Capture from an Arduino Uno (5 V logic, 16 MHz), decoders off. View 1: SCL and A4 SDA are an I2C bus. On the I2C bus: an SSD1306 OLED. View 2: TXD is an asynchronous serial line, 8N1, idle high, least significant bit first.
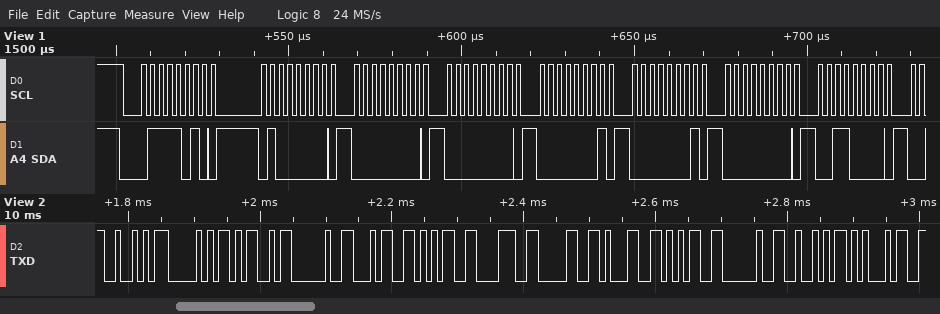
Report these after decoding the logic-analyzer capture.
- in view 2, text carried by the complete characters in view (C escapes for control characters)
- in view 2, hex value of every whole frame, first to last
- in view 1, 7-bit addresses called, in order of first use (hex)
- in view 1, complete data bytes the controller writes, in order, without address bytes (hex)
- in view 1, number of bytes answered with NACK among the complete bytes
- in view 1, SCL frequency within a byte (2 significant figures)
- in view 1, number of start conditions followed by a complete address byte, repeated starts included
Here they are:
"RPM 458015 RE"
52 50 4D 20 34 35 38 30 31 35 20 52 45
0x3D
40 00 00 01 01 00 30
0
400 kHz
1
